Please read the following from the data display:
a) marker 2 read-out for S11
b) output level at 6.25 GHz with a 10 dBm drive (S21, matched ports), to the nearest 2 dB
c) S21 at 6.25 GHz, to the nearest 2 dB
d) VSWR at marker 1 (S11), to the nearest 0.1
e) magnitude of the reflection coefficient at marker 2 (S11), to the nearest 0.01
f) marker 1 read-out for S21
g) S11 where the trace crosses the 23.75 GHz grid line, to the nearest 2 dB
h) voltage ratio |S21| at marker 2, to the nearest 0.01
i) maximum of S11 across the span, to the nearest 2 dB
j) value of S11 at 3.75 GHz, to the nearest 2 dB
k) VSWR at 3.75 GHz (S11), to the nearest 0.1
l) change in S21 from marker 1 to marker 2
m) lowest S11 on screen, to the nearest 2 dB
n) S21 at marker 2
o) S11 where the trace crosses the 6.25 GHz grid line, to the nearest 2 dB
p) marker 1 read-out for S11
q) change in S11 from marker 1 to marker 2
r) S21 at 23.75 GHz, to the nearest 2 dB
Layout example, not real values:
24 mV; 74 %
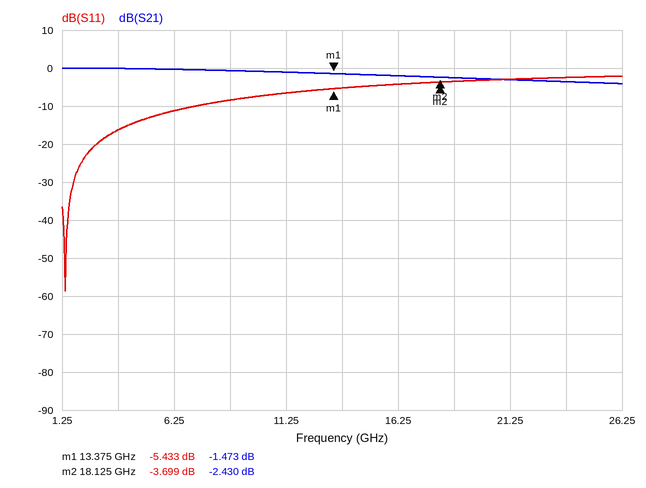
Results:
-3.699 dB; 10 dBm; 0 dB; 3.3; 0.65; -1.473 dB; -2 dB; 0.76; -2 dB; -16 dB; 1.4; -0.957 dB; -58 dB; -2.430 dB; -12 dB; -5.433 dB; 1.734 dB; -4 dB
